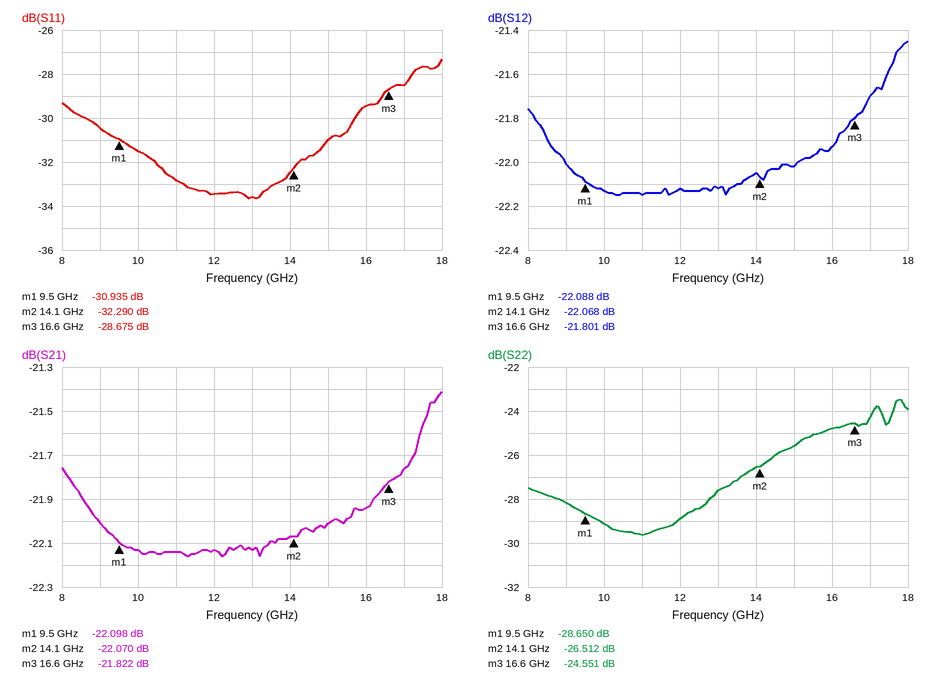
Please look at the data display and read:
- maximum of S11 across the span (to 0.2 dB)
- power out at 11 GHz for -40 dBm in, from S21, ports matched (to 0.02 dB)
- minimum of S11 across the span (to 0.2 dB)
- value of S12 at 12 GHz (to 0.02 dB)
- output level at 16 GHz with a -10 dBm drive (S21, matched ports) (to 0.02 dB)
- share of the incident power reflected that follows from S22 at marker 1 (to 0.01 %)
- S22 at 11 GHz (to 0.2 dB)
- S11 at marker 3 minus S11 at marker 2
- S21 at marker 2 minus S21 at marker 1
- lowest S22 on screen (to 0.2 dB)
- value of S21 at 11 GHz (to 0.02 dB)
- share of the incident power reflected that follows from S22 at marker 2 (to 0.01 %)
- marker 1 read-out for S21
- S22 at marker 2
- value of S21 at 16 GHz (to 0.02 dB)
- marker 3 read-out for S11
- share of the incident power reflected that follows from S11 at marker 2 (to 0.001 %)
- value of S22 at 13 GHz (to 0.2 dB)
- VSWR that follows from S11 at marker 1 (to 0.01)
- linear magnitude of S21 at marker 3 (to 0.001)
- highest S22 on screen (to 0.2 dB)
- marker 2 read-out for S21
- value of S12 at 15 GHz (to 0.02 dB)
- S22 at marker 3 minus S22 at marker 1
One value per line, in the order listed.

-27.4 dB
-62.14 dBm
-33.6 dB
-22.12 dB
-31.94 dBm
0.14 %
-29.6 dB
3.615 dB
0.028 dB
-29.6 dB
-22.14 dB
0.22 %
-22.098 dB
-26.512 dB
-21.94 dB
-28.675 dB
0.059 %
-27.6 dB
1.06
0.081
-23.4 dB
-22.070 dB
-22.02 dB
4.099 dB
